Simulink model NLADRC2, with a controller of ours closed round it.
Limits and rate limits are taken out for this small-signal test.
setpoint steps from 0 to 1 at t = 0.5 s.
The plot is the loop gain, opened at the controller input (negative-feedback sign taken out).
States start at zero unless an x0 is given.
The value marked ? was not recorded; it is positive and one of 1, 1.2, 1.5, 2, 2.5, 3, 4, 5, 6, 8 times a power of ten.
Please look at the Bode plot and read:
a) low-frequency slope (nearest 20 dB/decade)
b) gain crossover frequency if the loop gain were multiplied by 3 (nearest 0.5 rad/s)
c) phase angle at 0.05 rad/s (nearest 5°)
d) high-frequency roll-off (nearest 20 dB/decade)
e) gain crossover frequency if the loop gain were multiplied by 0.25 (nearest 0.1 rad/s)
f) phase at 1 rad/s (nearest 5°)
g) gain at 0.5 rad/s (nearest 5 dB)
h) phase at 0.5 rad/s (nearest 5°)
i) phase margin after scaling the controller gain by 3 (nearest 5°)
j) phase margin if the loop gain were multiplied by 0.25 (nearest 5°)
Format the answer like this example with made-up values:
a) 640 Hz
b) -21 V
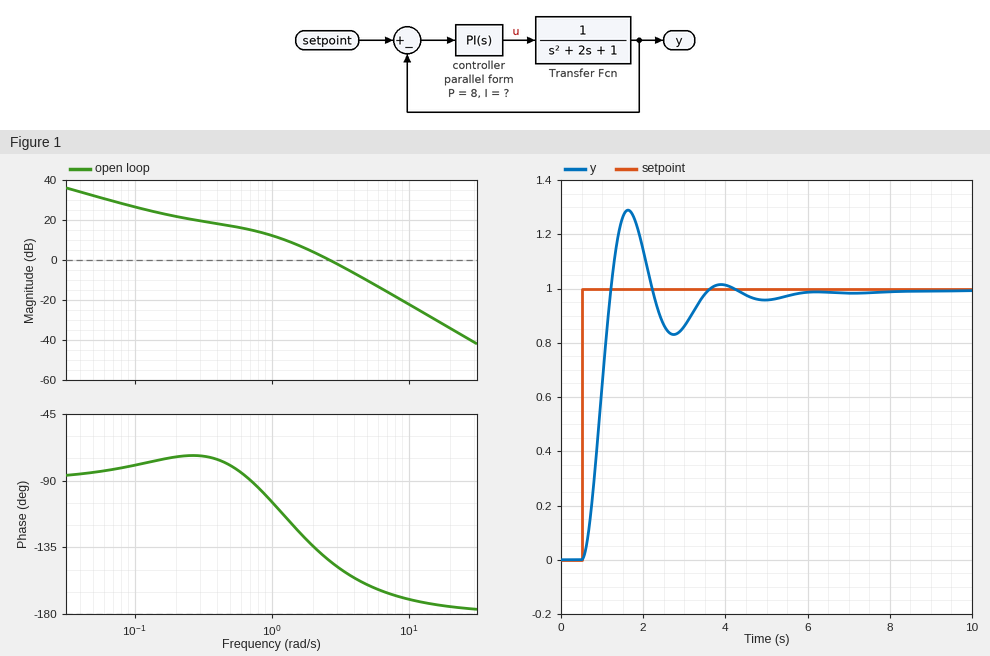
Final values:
a) -20 dB/decade
b) 5.0 rad/s
c) -85°
d) -40 dB/decade
e) 1.0 rad/s
f) -105°
g) 15 dB
h) -80°
i) 20°
j) 75°
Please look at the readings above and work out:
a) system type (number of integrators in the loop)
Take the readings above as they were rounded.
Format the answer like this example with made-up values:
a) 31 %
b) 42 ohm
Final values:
a) 1
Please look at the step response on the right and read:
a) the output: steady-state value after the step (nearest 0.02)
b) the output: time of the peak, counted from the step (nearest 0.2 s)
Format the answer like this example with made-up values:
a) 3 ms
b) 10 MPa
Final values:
a) 1.00
b) 1.2 s
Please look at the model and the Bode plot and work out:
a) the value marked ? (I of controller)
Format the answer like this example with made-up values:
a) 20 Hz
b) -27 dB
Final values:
a) 2
